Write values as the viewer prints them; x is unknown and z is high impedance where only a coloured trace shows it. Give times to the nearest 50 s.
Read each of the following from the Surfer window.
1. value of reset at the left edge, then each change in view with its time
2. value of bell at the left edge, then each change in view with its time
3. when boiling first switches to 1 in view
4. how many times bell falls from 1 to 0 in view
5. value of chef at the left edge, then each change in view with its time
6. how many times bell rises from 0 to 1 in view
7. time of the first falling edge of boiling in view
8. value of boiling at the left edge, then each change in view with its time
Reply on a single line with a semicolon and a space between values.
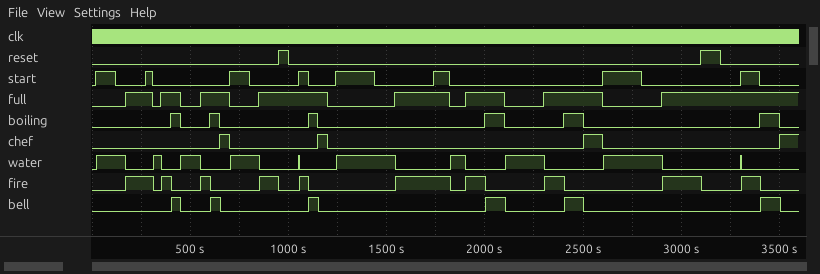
0, 1 at 950 s, 0 at 1000 s, 1 at 3100 s, 0 at 3200 s; 0, 1 at 400 s, 0 at 450 s, 1 at 600 s, 0 at 650 s, 1 at 1100 s, 0 at 1150 s, 1 at 2000 s, 0 at 2100 s, 1 at 2400 s, 0 at 2500 s, 1 at 3400 s, 0 at 3500 s; 400 s; 6; 0, 1 at 650 s, 0 at 700 s, 1 at 1150 s, 0 at 1200 s, 1 at 2500 s, 0 at 2600 s, 1 at 3500 s; 6; 450 s; 0, 1 at 400 s, 0 at 450 s, 1 at 600 s, 0 at 650 s, 1 at 1100 s, 0 at 1150 s, 1 at 2000 s, 0 at 2100 s, 1 at 2400 s, 0 at 2500 s, 1 at 3400 s, 0 at 3500 s
